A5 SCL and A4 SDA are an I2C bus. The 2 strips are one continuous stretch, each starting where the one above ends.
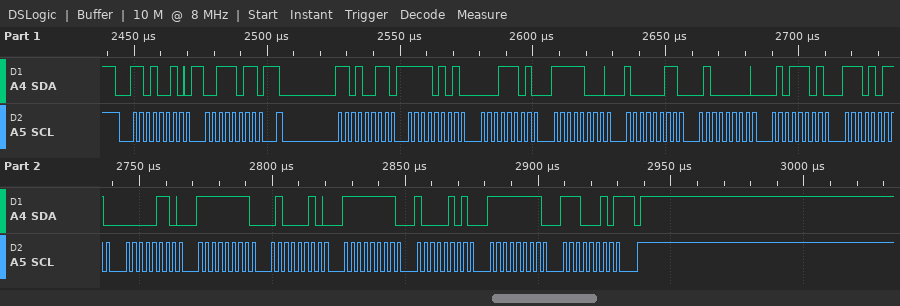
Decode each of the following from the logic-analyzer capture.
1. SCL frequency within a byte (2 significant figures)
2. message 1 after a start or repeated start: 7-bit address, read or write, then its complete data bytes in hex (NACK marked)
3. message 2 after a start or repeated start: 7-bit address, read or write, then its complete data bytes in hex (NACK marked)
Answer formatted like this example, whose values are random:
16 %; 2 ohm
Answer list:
400 kHz; 0x69 write: 3B; 0x69 read: F5 1D F8 83 40 5D EB 06 FF 42 FF 85 FF E2 NACK
